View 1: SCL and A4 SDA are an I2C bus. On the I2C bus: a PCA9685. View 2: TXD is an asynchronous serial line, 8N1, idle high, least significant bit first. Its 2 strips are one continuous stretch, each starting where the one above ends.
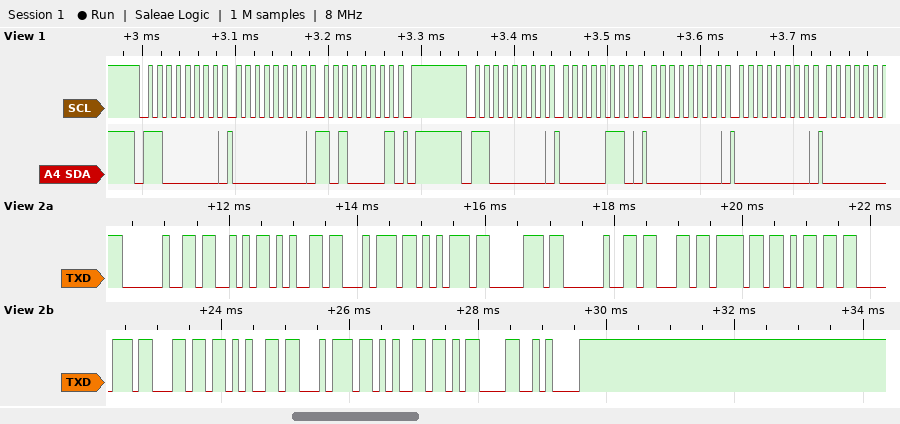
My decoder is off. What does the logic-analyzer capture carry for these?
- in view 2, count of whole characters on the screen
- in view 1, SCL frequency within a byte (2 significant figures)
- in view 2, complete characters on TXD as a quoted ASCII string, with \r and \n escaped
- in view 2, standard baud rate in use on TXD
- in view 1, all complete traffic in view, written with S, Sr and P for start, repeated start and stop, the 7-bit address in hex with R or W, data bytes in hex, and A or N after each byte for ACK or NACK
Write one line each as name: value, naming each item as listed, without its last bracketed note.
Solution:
in view 2, count of whole characters on the screen: 17
in view 1, SCL frequency within a byte: 100 kHz
in view 2, complete characters on TXD as a quoted ASCII string, with \r and \n escaped: " Setup complete\r\n"
in view 2, standard baud rate in use on TXD: 9600 baud
in view 1, all complete traffic in view, written with S, Sr and P for start, repeated start and stop, the 7-bit address in hex with R or W, data bytes in hex, and A or N after each byte for ACK or NACK: S 60W A 00 A A1 A P S 60W A 06 A 00 A 00 A
